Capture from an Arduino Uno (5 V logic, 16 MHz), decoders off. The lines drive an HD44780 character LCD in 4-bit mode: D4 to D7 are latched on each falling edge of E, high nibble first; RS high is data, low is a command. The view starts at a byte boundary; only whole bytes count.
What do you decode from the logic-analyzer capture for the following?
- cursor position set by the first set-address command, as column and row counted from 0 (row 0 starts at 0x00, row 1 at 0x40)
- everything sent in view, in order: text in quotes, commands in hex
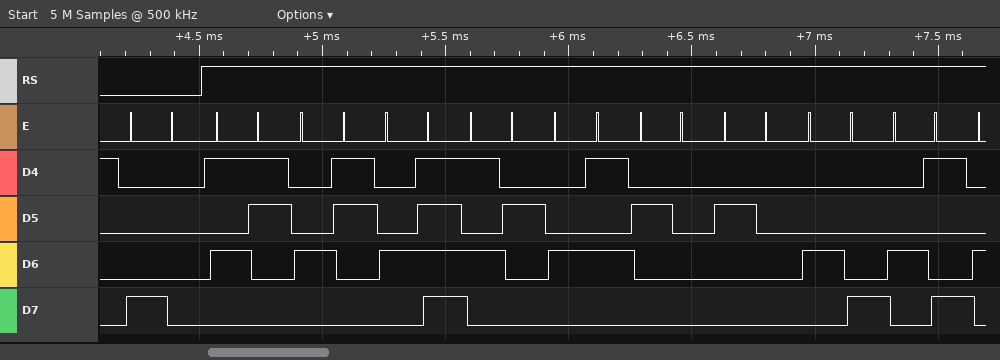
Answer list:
column 0, row 0
0x80 "SCORE  HI"
